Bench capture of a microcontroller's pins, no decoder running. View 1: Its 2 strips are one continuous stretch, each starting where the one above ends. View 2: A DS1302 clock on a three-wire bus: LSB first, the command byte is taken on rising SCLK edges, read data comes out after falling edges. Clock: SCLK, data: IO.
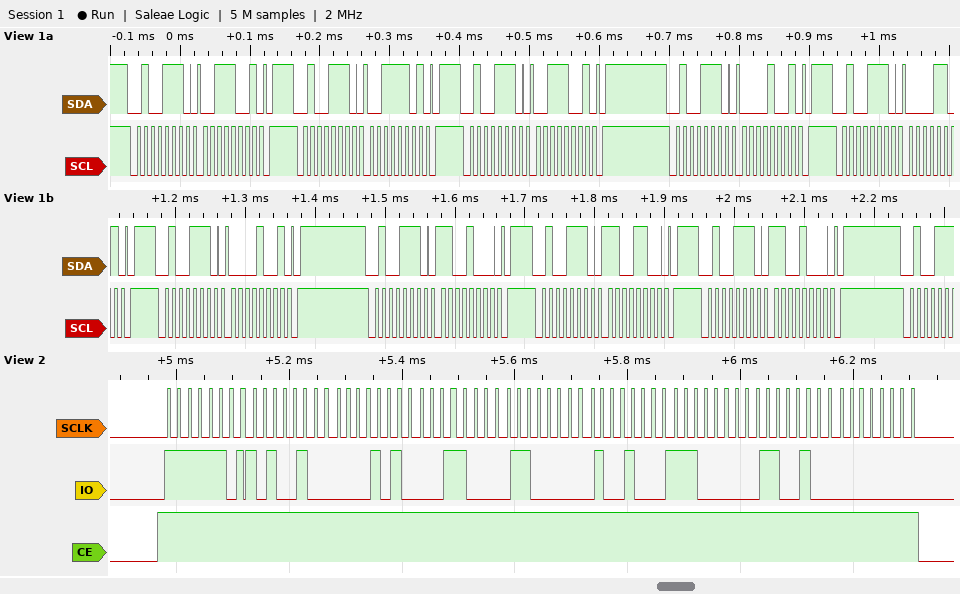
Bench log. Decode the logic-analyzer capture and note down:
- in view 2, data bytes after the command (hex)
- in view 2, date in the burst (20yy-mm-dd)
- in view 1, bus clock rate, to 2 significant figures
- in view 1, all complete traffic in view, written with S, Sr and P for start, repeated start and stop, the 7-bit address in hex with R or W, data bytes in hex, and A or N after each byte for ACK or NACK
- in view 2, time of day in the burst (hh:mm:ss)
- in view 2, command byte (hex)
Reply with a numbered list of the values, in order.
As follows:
1. 25 50 18 06 12 07 26 00
2. 2026-12-06
3. 100 kHz
4. S 27W A 39 A P S 27W A 3D A P S 27W A 39 A P S 27W A 09 A P S 27W A 0D A P S 27W A 09 A P S 27W A C8 A P S 27W A CC A P S 27W A C8 A P
5. 18:50:25
6. 0xBF
